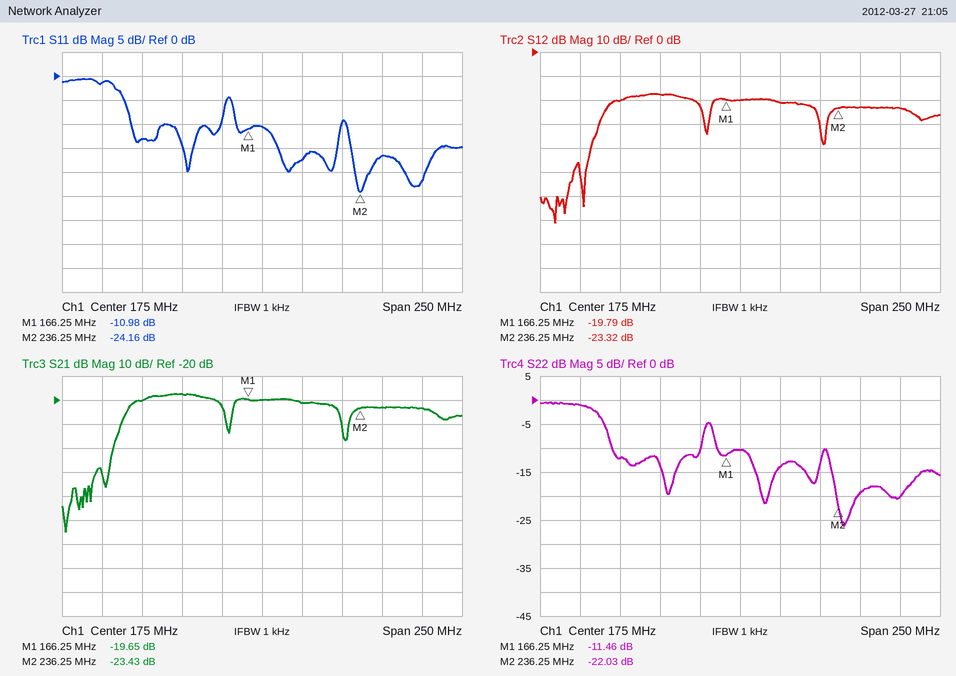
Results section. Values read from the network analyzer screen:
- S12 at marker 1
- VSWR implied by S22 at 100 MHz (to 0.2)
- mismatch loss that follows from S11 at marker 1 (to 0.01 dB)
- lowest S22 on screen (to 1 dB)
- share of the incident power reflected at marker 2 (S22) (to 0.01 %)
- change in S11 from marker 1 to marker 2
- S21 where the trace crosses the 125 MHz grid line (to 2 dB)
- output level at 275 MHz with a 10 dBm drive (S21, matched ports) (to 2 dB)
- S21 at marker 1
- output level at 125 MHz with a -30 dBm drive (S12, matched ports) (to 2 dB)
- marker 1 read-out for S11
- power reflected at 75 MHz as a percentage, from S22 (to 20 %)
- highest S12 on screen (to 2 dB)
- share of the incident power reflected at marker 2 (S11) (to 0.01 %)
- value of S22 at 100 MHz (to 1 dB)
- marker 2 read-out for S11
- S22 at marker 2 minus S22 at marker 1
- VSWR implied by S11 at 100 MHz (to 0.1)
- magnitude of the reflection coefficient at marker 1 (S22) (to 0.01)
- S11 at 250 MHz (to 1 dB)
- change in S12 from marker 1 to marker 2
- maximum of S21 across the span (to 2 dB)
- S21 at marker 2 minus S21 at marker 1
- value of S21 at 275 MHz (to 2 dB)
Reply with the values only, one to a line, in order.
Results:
-19.79 dB
1.6
0.36 dB
-26 dB
0.63 %
-13.18 dB
-18 dB
-14 dBm
-19.65 dB
-48 dBm
-10.98 dB
80 %
-18 dB
0.38 %
-12 dB
-24.16 dB
-10.57 dB
1.6
0.27
-17 dB
-3.53 dB
-18 dB
-3.78 dB
-24 dB
